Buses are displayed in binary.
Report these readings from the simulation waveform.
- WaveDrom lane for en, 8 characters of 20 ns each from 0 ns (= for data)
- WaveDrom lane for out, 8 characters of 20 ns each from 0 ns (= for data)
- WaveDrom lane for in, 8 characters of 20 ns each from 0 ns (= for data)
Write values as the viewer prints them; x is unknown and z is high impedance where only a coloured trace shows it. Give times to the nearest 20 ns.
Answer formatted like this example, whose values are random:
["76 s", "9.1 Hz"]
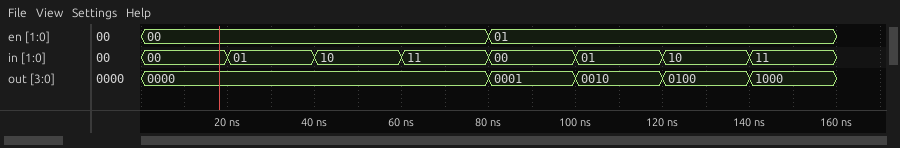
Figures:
["{name: 'en', wave: '=...=...', data: '00 01'}", "{name: 'out', wave: '=...====', data: '0000 0001 0010 0100 1000'}", "{name: 'in', wave: '========', data: '00 01 10 11 00 01 10 11'}"]
